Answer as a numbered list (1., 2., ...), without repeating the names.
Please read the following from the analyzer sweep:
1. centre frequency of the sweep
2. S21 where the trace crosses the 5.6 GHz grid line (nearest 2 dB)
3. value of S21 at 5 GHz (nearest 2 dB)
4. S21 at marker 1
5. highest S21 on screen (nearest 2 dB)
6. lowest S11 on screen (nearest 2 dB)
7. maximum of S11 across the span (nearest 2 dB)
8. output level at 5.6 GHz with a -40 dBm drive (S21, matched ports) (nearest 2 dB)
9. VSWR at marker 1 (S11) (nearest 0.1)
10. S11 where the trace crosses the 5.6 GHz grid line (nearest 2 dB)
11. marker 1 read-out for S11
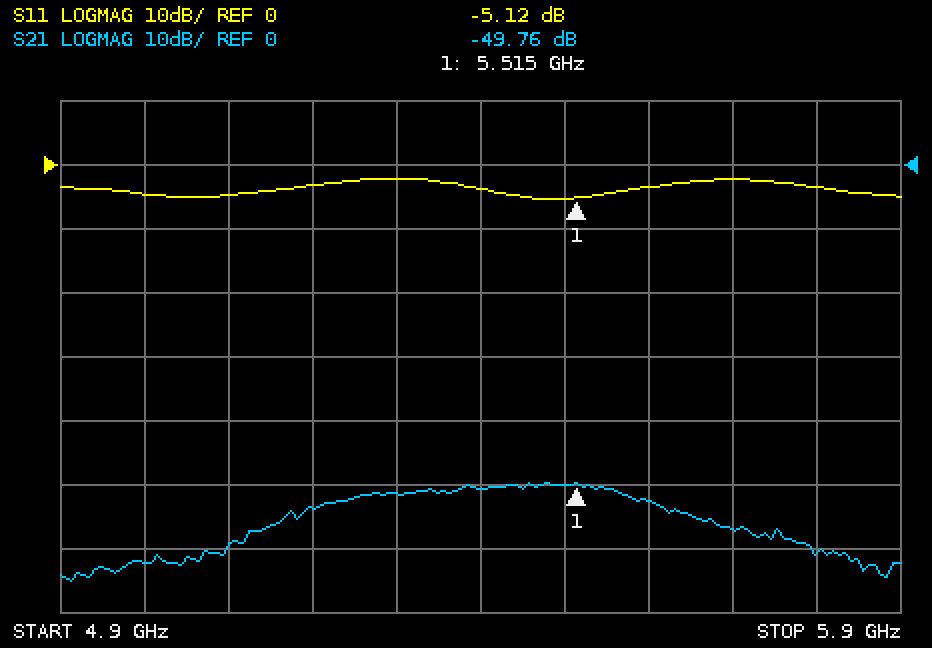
1. 5.4 GHz
2. -52 dB
3. -62 dB
4. -49.76 dB
5. -50 dB
6. -6 dB
7. -2 dB
8. -92 dBm
9. 3.5
10. -4 dB
11. -5.12 dB
